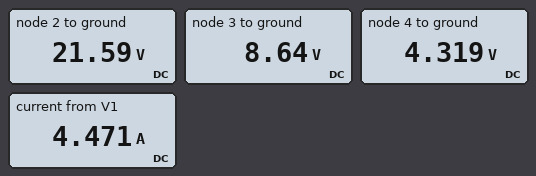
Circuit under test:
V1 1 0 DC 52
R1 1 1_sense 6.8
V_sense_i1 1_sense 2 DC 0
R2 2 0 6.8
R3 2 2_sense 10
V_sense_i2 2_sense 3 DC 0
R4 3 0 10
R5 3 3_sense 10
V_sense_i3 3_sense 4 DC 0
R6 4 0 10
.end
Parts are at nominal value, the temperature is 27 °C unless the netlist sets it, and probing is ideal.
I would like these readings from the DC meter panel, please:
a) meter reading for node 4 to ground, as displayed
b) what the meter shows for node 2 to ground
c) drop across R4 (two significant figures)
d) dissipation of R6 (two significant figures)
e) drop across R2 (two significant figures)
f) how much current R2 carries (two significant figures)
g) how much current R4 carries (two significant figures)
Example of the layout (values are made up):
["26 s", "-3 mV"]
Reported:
["4.319 V", "21.59 V", "8.6 V", "1.9 W", "22 V", "3.2 A", "860 mA"]
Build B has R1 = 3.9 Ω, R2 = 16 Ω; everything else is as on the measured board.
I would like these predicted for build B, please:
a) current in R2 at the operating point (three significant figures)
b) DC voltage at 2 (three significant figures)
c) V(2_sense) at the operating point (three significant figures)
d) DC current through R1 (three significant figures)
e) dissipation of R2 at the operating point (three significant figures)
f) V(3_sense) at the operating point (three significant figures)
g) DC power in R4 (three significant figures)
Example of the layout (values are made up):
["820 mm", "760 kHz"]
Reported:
["2.20 A", "35.2 V", "14.1 V", "4.31 A", "77.4 W", "7.04 V", "19.8 W"]
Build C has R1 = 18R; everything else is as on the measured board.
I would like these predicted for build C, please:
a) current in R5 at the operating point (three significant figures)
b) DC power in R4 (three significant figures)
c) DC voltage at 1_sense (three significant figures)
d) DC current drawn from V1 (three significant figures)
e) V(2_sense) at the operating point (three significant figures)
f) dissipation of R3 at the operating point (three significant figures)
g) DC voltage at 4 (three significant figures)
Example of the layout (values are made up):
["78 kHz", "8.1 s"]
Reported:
["220 mA", "1.94 W", "11.0 V", "2.28 A", "4.40 V", "4.36 W", "2.20 V"]
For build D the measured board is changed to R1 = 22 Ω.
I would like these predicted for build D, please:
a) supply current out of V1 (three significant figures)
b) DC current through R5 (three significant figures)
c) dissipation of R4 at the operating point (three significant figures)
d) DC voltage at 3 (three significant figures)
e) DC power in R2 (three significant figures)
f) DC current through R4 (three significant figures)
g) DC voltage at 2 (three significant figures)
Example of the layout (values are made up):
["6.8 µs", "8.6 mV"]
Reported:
["1.94 A", "187 mA", "1.40 W", "3.74 V", "12.9 W", "374 mA", "9.36 V"]
